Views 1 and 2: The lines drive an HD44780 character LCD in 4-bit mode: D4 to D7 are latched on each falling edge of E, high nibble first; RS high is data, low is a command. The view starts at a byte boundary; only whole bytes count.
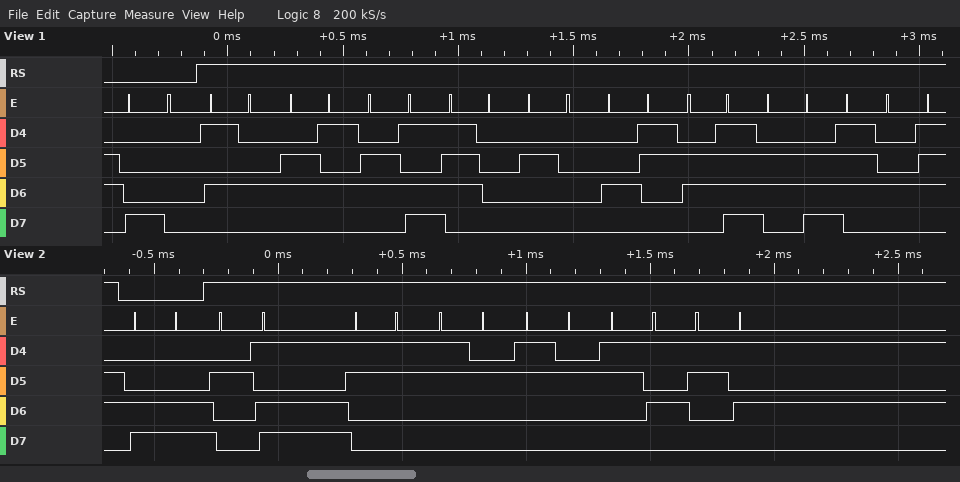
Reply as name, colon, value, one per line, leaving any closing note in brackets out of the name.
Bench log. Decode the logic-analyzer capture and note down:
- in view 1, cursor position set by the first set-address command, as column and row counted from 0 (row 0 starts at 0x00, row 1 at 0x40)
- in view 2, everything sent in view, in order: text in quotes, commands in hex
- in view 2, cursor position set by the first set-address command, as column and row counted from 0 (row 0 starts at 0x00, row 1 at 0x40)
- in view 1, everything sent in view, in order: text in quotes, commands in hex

in view 1, cursor position set by the first set-address command, as column and row counted from 0: column 0, row 0
in view 2, everything sent in view, in order: text in quotes, commands in hex: 0xCC "-32255"
in view 2, cursor position set by the first set-address command, as column and row counted from 0: column 12, row 1
in view 1, everything sent in view, in order: text in quotes, commands in hex: 0x80 "Temp Cont"
